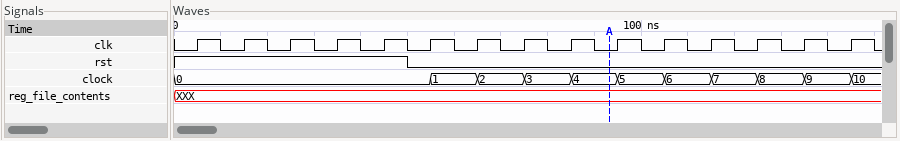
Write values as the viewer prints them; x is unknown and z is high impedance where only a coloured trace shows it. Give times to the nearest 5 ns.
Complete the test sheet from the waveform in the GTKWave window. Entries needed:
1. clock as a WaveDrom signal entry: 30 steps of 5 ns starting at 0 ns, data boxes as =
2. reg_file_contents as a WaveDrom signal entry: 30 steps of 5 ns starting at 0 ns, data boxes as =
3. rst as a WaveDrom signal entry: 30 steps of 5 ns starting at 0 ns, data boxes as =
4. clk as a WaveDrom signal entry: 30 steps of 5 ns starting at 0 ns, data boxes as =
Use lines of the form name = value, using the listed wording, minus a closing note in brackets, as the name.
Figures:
clock as a WaveDrom signal entry: 30 steps of 5 ns starting at 0 ns, data boxes as = = {name: 'clock', wave: '=..........=.=.=.=.=.=.=.=.=.=', data: '0 1 2 3 4 5 6 7 8 9 10'}
reg_file_contents as a WaveDrom signal entry: 30 steps of 5 ns starting at 0 ns, data boxes as = = {name: 'reg_file_contents', wave: 'x.............................'}
rst as a WaveDrom signal entry: 30 steps of 5 ns starting at 0 ns, data boxes as = = {name: 'rst', wave: '1.........0...................'}
clk as a WaveDrom signal entry: 30 steps of 5 ns starting at 0 ns, data boxes as = = {name: 'clk', wave: '010101010101010101010101010101'}
